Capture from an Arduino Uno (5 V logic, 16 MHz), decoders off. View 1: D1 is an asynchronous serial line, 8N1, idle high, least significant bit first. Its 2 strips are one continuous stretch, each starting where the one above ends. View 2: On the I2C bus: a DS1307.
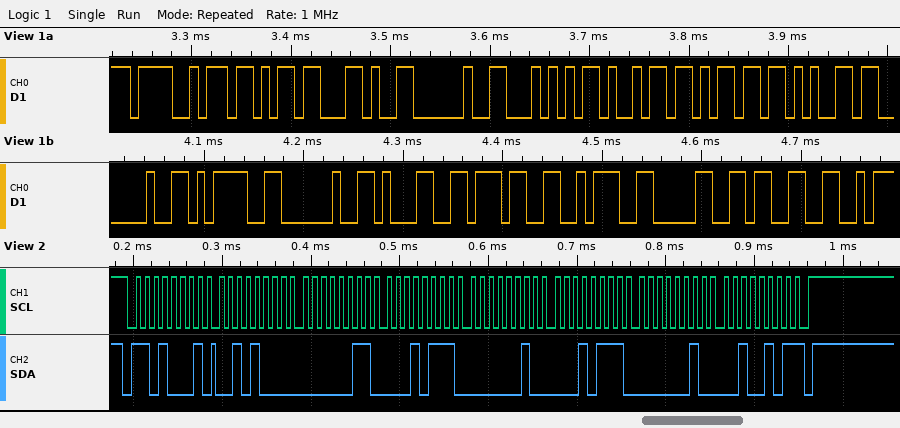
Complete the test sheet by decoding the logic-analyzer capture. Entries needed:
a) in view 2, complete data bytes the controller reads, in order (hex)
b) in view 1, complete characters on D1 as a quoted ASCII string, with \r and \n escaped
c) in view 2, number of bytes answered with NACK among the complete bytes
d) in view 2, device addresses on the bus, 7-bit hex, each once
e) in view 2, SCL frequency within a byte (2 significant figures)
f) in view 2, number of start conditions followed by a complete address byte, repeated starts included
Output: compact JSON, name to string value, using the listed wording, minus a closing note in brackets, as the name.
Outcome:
{"in view 2, complete data bytes the controller reads, in order": "28 03 17 02 17 02 25", "in view 1, complete characters on D1 as a quoted ASCII string, with \\r and \\n escaped": "\"Ok, Time = 17:03\"", "in view 2, number of bytes answered with NACK among the complete bytes": "1", "in view 2, device addresses on the bus, 7-bit hex, each once": "0x68", "in view 2, SCL frequency within a byte": "100 kHz", "in view 2, number of start conditions followed by a complete address byte, repeated starts included": "1"}
